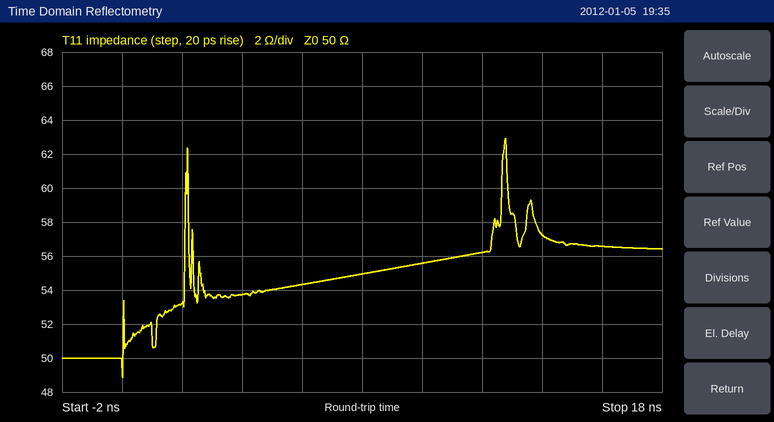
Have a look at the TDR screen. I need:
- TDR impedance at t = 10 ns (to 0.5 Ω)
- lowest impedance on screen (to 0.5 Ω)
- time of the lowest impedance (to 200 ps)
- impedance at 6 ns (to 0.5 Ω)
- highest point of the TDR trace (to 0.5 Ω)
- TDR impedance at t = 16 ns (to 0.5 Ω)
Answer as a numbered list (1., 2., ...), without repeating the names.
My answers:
1. 55.5 Ω
2. 49.0 Ω
3. 0.0 ns
4. 54.5 Ω
5. 63.0 Ω
6. 56.5 Ω
